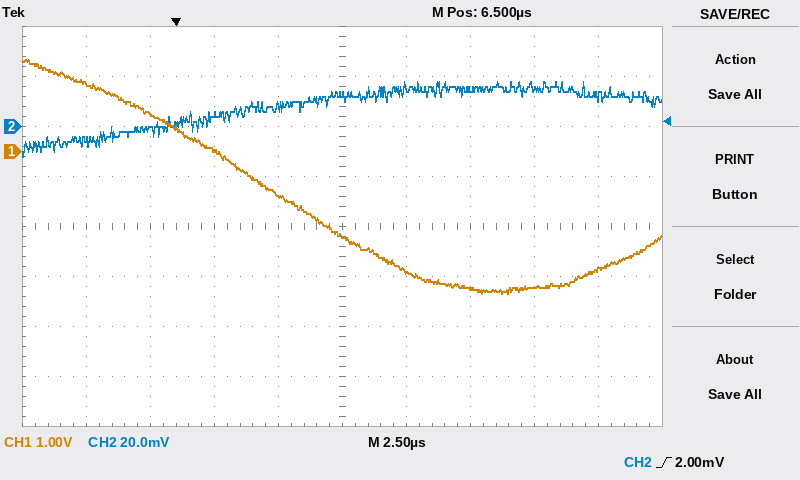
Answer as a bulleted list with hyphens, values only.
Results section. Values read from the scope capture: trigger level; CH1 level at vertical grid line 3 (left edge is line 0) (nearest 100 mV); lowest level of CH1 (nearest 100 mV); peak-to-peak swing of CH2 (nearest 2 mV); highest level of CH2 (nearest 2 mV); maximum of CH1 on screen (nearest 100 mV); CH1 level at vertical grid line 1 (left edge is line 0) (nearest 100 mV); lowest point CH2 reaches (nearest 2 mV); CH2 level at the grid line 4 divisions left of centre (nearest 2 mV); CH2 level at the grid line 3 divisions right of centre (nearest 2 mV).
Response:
- 2.00 mV
- 0.0 V
- -2.8 V
- 30 mV
- 18 mV
- 1.8 V
- 1.4 V
- -12 mV
- -6 mV
- 16 mV
